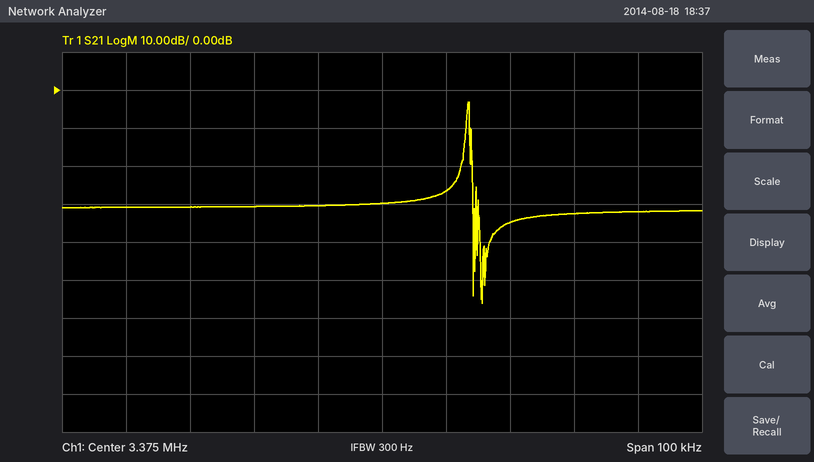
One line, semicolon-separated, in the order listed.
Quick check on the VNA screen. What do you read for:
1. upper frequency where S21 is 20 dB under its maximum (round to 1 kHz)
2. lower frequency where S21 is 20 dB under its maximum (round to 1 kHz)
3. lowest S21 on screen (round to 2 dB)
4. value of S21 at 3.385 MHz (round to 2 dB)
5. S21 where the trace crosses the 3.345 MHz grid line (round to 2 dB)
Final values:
3.389 MHz; 3.387 MHz; -56 dB; -26 dB; -30 dB
